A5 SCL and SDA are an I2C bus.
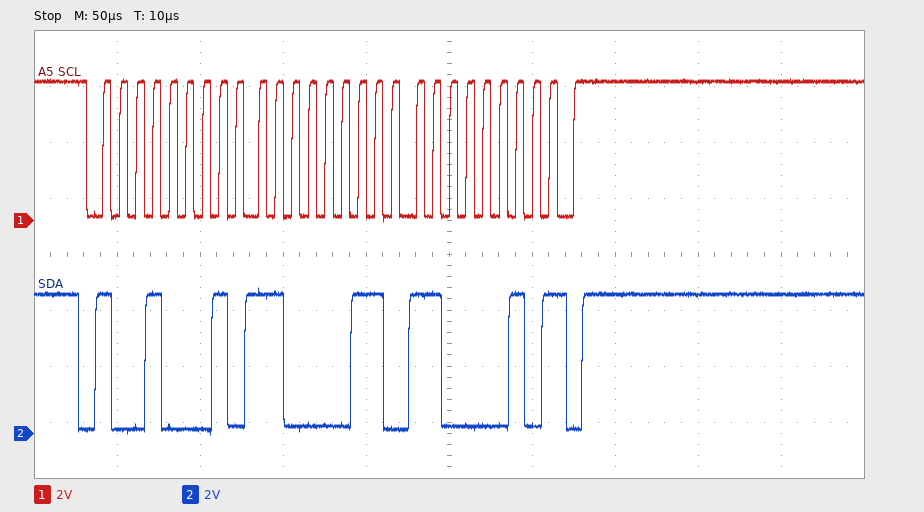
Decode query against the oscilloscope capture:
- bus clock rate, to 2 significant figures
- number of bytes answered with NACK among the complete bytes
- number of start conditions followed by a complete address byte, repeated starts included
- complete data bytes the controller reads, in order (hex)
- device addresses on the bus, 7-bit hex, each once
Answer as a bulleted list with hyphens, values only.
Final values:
- 100 kHz
- 1
- 1
- C3 C2
- 0x48
